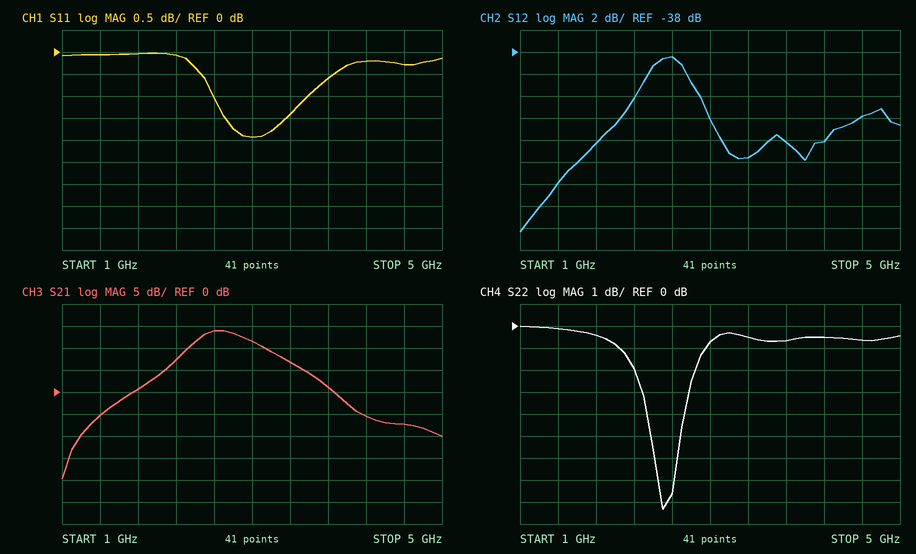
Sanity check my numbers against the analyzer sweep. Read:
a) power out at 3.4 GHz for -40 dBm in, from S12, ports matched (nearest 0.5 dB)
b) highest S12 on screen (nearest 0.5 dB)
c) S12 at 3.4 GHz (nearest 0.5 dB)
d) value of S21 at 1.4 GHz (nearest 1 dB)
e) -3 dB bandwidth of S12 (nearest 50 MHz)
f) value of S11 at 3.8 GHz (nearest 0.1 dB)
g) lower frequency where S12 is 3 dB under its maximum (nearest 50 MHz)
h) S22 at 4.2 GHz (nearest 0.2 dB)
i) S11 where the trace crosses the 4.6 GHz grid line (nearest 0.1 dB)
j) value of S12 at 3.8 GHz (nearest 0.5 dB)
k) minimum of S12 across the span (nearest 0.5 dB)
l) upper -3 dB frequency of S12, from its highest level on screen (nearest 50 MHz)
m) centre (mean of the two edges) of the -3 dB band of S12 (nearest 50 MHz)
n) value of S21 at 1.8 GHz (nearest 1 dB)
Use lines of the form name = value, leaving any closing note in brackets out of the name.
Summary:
power out at 3.4 GHz for -40 dBm in, from S12, ports matched = -87.5 dBm
highest S12 on screen = -38.5 dB
S12 at 3.4 GHz = -47.5 dB
value of S21 at 1.4 GHz = -5 dB
-3 dB bandwidth of S12 = 600 MHz
value of S11 at 3.8 GHz = -0.6 dB
lower frequency where S12 is 3 dB under its maximum = 2.25 GHz
S22 at 4.2 GHz = -0.6 dB
S11 where the trace crosses the 4.6 GHz grid line = -0.3 dB
value of S12 at 3.8 GHz = -46.0 dB
minimum of S12 across the span = -54.5 dB
upper -3 dB frequency of S12, from its highest level on screen = 2.85 GHz
centre (mean of the two edges) of the -3 dB band of S12 = 2.55 GHz
value of S21 at 1.8 GHz = 1 dB
